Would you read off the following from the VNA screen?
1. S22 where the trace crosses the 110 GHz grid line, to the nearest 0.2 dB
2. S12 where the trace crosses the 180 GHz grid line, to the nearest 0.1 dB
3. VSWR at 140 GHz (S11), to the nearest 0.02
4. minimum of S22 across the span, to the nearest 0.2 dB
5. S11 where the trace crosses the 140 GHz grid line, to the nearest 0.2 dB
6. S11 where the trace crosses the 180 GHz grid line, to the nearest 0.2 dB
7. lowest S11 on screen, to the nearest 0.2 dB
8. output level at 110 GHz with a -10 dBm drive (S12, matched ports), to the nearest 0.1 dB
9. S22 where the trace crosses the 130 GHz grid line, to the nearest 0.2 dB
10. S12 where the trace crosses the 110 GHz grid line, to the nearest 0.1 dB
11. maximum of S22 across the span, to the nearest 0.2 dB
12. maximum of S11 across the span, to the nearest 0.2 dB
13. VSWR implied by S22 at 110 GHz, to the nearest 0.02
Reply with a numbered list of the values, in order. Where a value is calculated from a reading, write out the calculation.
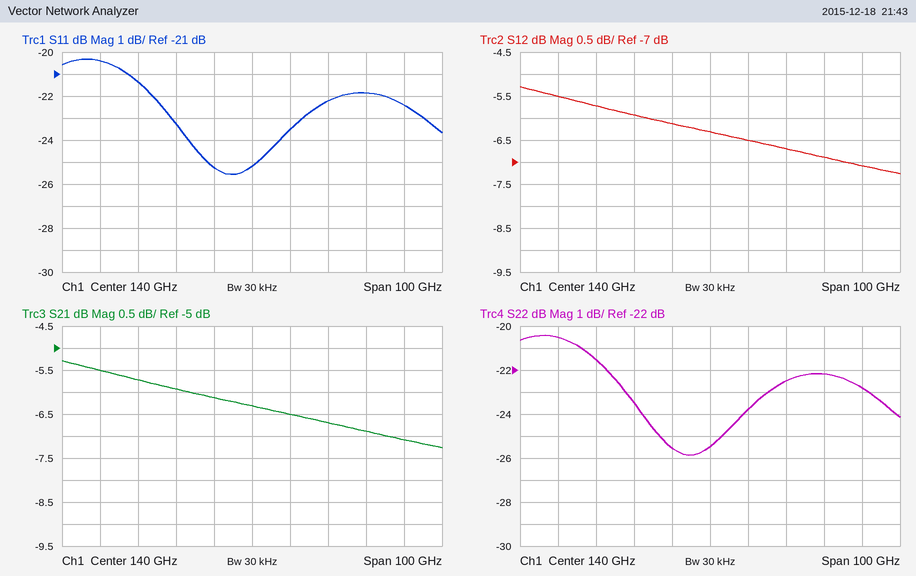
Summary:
1. -21.6 dB
2. -7.1 dB
3. |Γ| = 10^(-25.2/20) = 0.0550; VSWR = (1 + 0.0550)/(1 − 0.0550) ≈ 1.12
4. -25.8 dB
5. -25.2 dB
6. -22.4 dB
7. -25.6 dB
8. -10 dBm + (-5.7 dB) = -15.7 dBm
9. -25.6 dB
10. -5.7 dB
11. -20.4 dB
12. -20.4 dB
13. |Γ| = 10^(-21.6/20) = 0.0832; VSWR = (1 + 0.0832)/(1 − 0.0832) ≈ 1.18
